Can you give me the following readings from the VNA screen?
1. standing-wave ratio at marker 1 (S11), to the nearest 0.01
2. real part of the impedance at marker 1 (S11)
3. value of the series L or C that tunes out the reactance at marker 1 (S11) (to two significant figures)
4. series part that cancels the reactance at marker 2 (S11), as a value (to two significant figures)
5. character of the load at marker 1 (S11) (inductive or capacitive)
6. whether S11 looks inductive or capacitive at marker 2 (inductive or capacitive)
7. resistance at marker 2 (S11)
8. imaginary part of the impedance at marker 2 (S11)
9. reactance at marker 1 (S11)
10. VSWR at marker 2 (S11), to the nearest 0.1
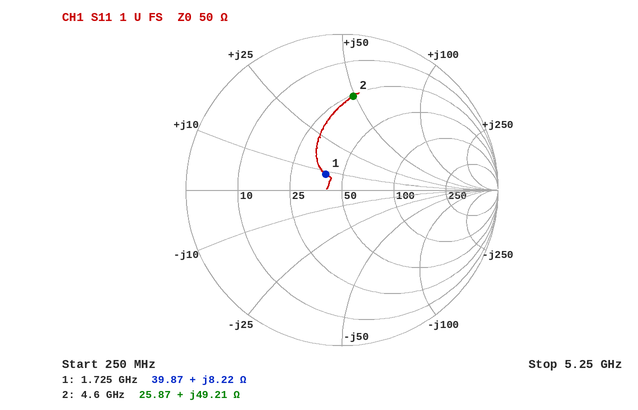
1.34
39.87 Ω
11 pF
700 fF
inductive
inductive
25.87 Ω
+49.21 Ω
+8.22 Ω
4.1
